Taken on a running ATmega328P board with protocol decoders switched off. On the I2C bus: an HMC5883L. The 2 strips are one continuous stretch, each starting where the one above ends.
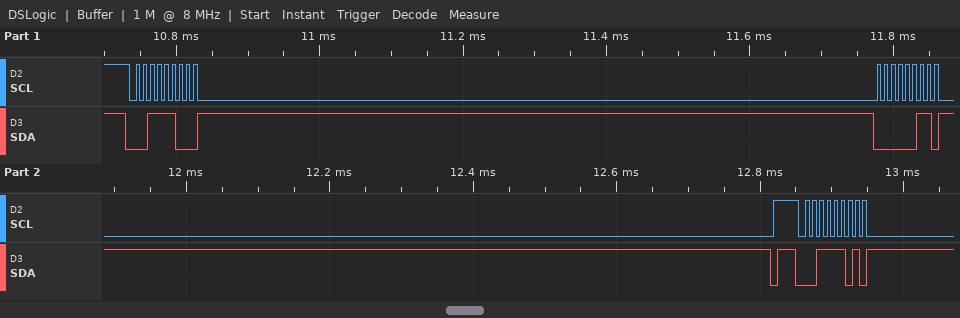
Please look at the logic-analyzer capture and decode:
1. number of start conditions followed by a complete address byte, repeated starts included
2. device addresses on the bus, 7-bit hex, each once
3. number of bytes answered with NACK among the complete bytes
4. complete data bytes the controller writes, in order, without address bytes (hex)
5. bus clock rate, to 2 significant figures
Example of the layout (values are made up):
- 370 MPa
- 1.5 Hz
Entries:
- 2
- 0x1E
- 0
- 03
- 100 kHz
